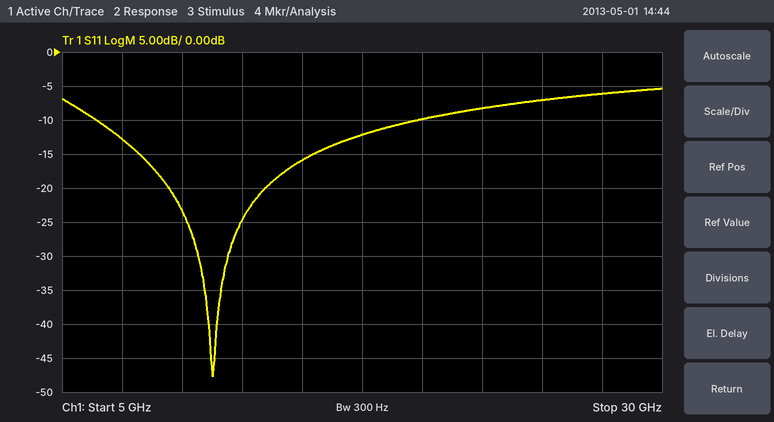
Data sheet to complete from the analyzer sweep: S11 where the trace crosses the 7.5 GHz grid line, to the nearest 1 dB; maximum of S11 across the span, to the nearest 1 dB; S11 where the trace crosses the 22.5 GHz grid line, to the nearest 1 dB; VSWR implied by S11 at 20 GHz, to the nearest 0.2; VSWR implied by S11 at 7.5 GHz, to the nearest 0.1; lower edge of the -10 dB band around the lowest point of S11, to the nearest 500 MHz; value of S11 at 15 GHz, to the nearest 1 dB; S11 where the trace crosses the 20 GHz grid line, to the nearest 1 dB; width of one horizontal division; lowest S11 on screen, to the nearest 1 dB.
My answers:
-13 dB
-5 dB
-8 dB
2.0
1.6
6.5 GHz
-16 dB
-10 dB
2.5 GHz
-48 dB
